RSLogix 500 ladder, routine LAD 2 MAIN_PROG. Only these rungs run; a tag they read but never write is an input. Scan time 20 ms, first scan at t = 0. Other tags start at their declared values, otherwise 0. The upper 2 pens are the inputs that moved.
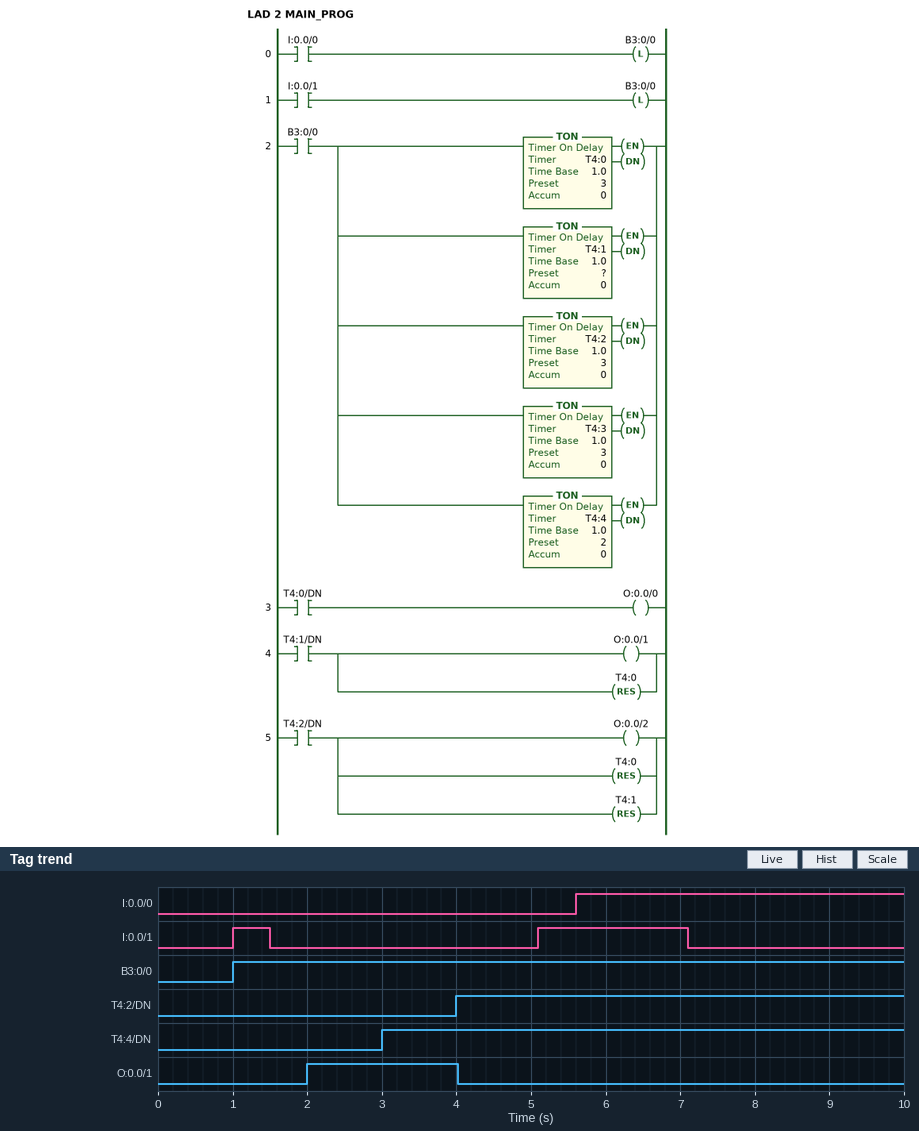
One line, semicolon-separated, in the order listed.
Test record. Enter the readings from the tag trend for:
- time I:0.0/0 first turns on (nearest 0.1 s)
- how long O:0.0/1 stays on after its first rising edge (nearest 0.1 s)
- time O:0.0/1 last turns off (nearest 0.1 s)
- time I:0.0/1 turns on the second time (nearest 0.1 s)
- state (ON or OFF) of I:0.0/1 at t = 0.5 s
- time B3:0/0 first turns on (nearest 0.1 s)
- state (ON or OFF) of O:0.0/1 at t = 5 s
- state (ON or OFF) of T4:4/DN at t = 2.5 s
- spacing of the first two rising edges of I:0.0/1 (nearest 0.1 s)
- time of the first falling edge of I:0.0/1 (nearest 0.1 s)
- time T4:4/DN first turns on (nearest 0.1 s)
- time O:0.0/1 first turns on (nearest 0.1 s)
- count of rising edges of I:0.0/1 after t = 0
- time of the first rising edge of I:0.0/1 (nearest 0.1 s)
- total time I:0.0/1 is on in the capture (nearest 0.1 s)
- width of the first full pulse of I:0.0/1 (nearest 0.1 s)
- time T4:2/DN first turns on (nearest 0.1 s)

5.6 s; 2.0 s; 4.0 s; 5.1 s; OFF; 1.0 s; OFF; OFF; 4.1 s; 1.5 s; 3.0 s; 2.0 s; 2; 1.0 s; 2.5 s; 0.5 s; 4.0 s
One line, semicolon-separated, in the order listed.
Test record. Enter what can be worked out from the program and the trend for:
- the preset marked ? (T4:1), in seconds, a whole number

1 s
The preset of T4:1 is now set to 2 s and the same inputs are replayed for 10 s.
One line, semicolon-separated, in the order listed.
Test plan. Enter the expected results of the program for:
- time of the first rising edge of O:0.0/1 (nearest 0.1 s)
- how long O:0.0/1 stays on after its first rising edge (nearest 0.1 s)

3.0 s; 1.0 s
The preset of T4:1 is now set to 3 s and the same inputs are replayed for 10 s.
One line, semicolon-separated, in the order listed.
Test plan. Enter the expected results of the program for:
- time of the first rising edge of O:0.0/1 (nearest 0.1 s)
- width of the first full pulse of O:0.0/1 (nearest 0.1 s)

4.0 s; 0.0 s
